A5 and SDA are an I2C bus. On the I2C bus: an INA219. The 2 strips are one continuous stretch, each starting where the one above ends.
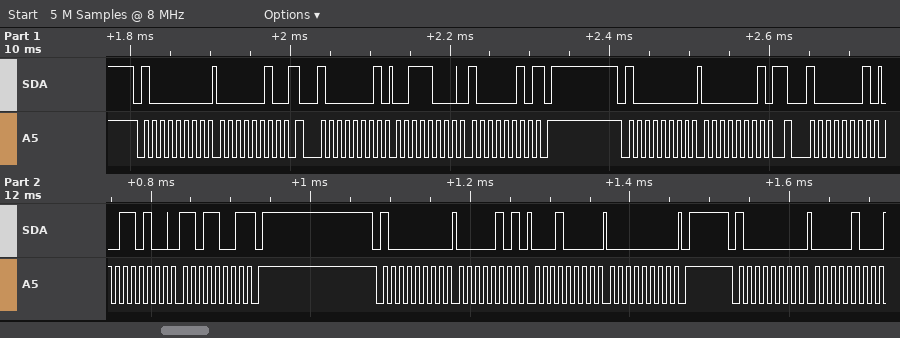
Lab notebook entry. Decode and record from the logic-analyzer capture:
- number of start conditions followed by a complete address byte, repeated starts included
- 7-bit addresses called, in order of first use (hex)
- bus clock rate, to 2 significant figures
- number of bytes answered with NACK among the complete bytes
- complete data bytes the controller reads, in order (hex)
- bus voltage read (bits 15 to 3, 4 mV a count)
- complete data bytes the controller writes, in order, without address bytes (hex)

6
0x40
100 kHz
2
38 82 34 D9
7.232 V
02 01 05 10 00 04
